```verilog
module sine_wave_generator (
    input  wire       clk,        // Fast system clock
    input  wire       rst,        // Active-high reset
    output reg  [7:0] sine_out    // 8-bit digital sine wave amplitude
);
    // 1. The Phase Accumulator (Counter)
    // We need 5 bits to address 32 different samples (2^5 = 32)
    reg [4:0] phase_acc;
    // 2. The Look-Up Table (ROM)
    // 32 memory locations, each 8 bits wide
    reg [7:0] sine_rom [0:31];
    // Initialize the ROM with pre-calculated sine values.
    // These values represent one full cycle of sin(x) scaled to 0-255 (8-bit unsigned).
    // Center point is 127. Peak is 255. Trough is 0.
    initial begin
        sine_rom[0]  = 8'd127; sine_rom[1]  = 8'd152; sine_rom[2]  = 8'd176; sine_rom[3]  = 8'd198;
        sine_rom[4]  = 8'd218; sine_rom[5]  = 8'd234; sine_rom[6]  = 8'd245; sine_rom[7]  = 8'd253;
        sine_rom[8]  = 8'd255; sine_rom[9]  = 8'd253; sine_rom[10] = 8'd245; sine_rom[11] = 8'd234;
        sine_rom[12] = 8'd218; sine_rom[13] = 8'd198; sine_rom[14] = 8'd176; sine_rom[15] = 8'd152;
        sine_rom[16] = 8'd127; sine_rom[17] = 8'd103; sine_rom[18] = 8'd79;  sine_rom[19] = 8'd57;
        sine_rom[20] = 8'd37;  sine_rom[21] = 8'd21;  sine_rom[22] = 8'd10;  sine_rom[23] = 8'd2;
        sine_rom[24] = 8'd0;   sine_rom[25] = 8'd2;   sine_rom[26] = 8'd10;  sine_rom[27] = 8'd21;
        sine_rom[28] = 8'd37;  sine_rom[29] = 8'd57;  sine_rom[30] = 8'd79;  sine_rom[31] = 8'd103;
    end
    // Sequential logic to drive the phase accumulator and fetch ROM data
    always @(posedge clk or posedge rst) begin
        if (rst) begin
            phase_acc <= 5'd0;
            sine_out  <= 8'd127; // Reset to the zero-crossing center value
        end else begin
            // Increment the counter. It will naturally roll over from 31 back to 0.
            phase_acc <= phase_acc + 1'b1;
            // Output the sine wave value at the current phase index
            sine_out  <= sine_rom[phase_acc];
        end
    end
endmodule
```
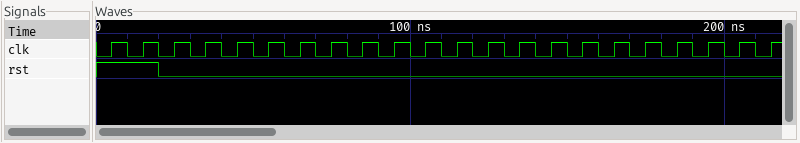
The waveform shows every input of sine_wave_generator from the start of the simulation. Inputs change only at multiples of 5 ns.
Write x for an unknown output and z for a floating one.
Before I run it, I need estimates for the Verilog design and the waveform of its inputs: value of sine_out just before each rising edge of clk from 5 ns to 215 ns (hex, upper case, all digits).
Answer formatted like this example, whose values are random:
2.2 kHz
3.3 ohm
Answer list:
7F, 7F, 7F, 7F, 98, B0, C6, DA, EA, F5, FD, FF, FD, F5, EA, DA, C6, B0, 98, 7F, 67, 4F
